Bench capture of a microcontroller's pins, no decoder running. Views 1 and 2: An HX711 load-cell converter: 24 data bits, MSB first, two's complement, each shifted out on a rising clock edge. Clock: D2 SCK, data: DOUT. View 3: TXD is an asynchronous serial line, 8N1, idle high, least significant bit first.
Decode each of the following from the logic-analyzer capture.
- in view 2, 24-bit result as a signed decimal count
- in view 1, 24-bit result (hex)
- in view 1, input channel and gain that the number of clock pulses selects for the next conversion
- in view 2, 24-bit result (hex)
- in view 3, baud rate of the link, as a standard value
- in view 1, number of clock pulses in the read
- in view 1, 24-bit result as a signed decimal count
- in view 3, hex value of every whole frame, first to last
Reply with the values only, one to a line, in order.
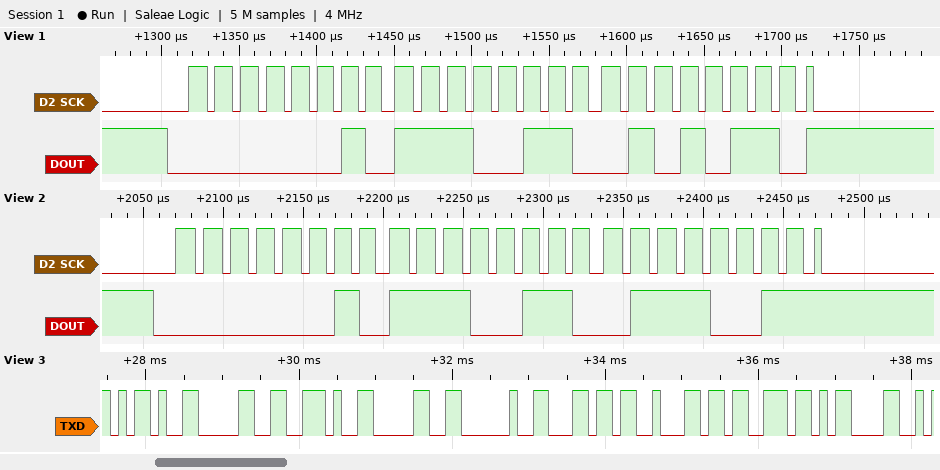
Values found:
190067
0x02E656
channel A, gain 128
0x02E673
9600 baud
25
190038
2D 30 2E 30 20 6C 62 73 0D
